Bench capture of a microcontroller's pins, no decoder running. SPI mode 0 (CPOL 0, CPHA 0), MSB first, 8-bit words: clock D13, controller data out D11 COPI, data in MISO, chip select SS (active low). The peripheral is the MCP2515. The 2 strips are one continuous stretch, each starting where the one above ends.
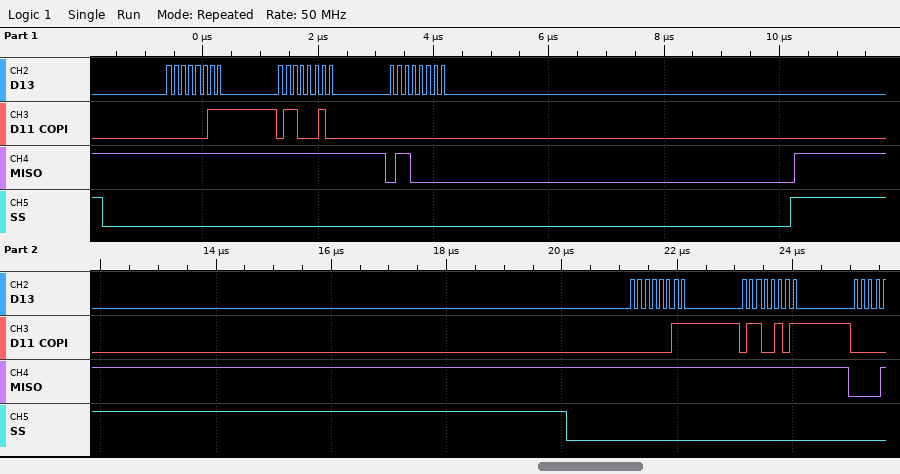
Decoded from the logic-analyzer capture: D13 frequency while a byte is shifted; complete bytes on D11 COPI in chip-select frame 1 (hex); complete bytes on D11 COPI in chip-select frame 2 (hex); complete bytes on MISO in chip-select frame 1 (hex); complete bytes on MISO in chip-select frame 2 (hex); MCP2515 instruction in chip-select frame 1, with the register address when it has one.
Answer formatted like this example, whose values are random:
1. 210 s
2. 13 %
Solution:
1. 8 MHz
2. 0x03 0x62 0x00
3. 0x03 0x65
4. 0xFF 0xFF 0x60
5. 0xFF 0xFF
6. READ 0x62
